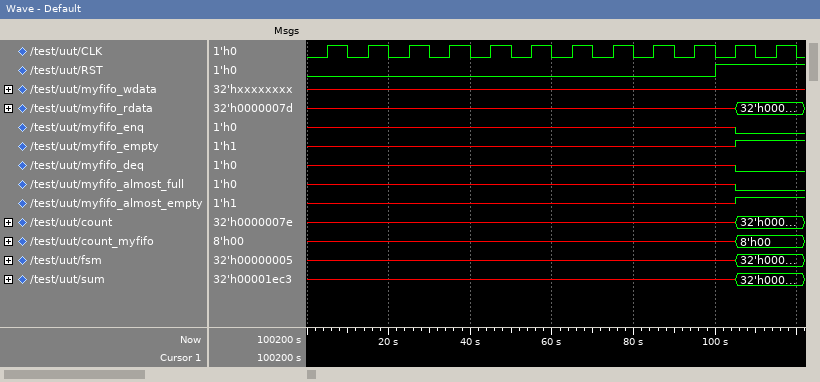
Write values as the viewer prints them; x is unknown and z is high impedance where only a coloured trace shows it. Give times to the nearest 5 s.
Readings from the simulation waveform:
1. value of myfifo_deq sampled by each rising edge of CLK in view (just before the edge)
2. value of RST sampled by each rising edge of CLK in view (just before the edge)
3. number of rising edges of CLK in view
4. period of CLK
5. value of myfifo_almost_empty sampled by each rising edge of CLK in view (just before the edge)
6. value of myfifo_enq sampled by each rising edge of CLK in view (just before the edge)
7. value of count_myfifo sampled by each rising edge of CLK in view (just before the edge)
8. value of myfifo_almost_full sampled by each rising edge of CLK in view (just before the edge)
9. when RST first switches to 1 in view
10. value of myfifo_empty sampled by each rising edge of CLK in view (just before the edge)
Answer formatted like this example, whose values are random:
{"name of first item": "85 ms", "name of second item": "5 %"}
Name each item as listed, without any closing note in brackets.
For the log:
{"value of myfifo_deq sampled by each rising edge of CLK in view": "x x x x x x x x x x x 0", "value of RST sampled by each rising edge of CLK in view": "0 0 0 0 0 0 0 0 0 0 1 1", "number of rising edges of CLK in view": "12", "period of CLK": "10 s", "value of myfifo_almost_empty sampled by each rising edge of CLK in view": "x x x x x x x x x x x 1", "value of myfifo_enq sampled by each rising edge of CLK in view": "x x x x x x x x x x x 0", "value of count_myfifo sampled by each rising edge of CLK in view": "x, x, x, x, x, x, x, x, x, x, x, 8'h00", "value of myfifo_almost_full sampled by each rising edge of CLK in view": "x x x x x x x x x x x 0", "when RST first switches to 1 in view": "100 s", "value of myfifo_empty sampled by each rising edge of CLK in view": "x x x x x x x x x x x 1"}
